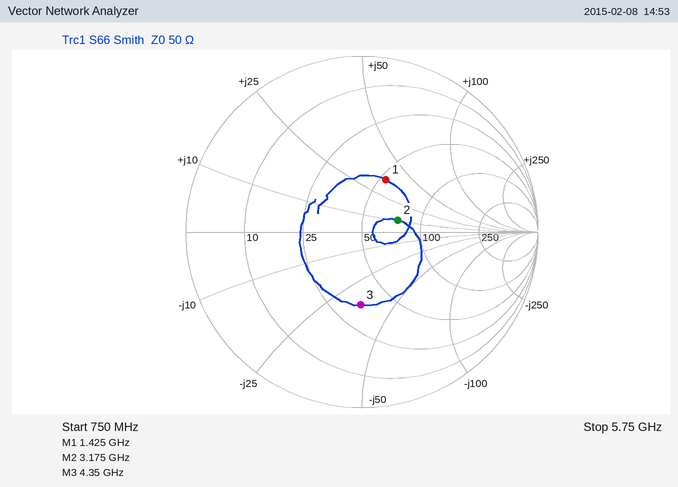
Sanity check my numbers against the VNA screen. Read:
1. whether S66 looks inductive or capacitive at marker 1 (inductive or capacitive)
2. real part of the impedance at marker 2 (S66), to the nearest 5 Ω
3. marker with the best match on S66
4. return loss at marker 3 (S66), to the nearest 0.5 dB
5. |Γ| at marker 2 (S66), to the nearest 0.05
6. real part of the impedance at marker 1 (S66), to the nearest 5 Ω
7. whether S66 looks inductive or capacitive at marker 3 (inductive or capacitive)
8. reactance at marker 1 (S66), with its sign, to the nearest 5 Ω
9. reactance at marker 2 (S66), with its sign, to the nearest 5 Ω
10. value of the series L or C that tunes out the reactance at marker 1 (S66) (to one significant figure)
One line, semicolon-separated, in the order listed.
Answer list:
inductive; 75 Ω; marker 2; 7.5 dB; 0.20; 55 Ω; capacitive; +35 Ω; +10 Ω; 3 pF
